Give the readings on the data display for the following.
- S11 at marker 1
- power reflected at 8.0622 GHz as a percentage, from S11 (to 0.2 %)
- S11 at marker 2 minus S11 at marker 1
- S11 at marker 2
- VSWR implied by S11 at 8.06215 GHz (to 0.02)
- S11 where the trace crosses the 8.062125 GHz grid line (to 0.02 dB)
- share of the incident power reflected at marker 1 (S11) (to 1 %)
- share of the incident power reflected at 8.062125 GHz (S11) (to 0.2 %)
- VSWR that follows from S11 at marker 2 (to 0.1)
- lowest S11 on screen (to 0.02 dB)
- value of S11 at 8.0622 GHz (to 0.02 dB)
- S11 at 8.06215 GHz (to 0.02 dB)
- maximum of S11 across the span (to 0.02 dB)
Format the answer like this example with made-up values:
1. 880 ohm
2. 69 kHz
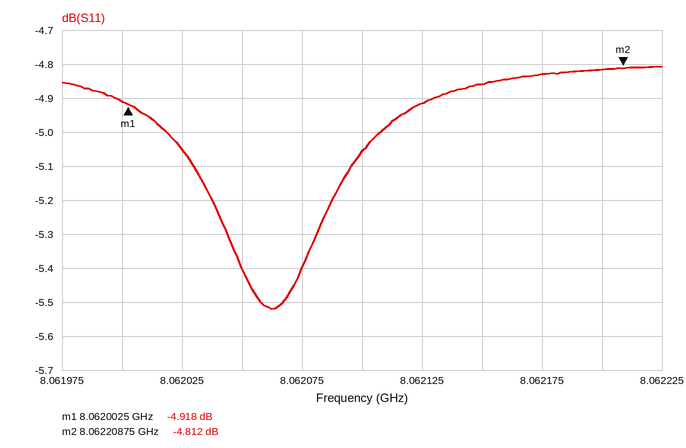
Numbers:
1. -4.918 dB
2. 33.0 %
3. 0.106 dB
4. -4.812 dB
5. 3.66
6. -4.92 dB
7. 32 %
8. 32.2 %
9. 3.7
10. -5.52 dB
11. -4.82 dB
12. -4.86 dB
13. -4.80 dB
